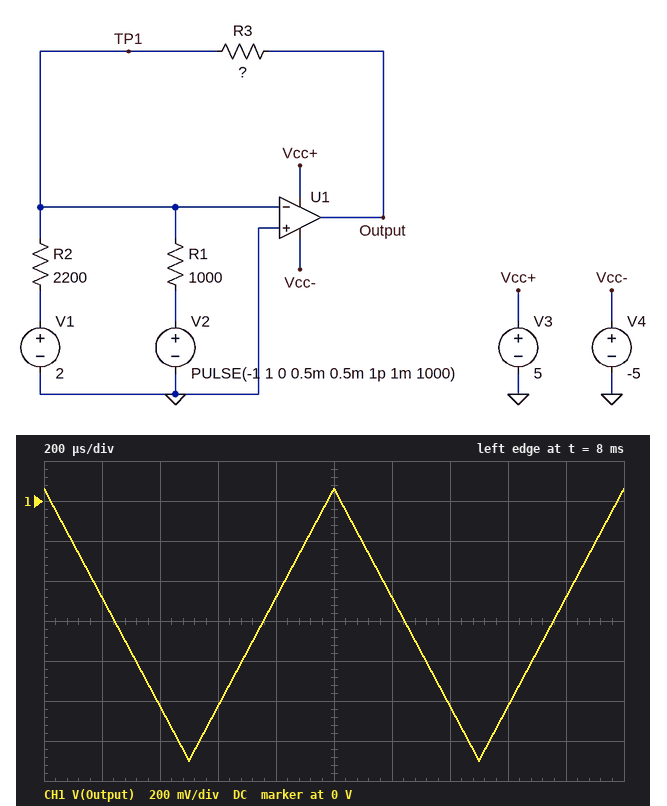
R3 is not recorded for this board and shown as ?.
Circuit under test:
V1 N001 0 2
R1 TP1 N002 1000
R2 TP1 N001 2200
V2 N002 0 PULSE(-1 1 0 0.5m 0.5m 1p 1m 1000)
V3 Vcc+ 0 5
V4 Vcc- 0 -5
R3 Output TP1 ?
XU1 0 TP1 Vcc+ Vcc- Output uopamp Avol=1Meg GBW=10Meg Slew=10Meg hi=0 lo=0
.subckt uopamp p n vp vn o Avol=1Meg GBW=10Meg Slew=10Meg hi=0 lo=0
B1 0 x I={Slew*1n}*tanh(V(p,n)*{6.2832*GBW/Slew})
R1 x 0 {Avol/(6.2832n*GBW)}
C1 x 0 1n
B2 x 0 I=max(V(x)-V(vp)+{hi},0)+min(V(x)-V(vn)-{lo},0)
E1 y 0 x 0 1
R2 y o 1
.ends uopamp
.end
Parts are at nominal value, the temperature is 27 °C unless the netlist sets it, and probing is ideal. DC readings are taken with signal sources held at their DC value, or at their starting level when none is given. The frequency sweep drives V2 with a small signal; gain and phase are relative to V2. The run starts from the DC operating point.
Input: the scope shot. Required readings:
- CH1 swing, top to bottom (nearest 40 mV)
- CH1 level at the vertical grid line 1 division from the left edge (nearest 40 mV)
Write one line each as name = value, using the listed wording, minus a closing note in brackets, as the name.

CH1 swing, top to bottom = 1.36 V
CH1 level at the vertical grid line 1 division from the left edge = -480 mV
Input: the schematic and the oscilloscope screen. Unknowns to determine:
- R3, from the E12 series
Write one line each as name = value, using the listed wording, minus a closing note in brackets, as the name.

R3, from the E12 series = 680 Ω
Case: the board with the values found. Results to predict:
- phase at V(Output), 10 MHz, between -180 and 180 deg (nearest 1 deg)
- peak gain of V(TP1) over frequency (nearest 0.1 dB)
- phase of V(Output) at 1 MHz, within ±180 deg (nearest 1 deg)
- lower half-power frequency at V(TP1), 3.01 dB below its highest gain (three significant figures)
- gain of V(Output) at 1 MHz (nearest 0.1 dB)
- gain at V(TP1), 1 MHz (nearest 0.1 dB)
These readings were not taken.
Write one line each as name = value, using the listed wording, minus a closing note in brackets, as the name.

phase at V(Output), 10 MHz, between -180 and 180 deg = 117 deg
peak gain of V(TP1) over frequency = -9.3 dB
phase of V(Output) at 1 MHz, within ±180 deg = 169 deg
lower half-power frequency at V(TP1), 3.01 dB below its highest gain = 5.02 MHz
gain of V(Output) at 1 MHz = -3.5 dB
gain at V(TP1), 1 MHz = -23.5 dB
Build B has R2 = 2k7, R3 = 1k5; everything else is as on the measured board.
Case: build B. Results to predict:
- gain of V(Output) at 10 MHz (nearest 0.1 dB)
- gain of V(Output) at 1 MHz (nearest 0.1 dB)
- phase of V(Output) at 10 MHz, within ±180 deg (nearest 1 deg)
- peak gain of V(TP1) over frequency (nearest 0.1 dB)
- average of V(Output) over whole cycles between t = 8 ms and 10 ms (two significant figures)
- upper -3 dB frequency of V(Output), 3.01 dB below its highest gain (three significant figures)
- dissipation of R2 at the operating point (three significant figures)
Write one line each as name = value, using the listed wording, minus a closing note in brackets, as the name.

gain of V(Output) at 10 MHz = -6.6 dB
gain of V(Output) at 1 MHz = 3.1 dB
phase of V(Output) at 10 MHz, within ±180 deg = 108 deg
peak gain of V(TP1) over frequency = -6.2 dB
average of V(Output) over whole cycles between t = 8 ms and 10 ms = -1.1 V
upper -3 dB frequency of V(Output), 3.01 dB below its highest gain = 3.27 MHz
dissipation of R2 at the operating point = 1.48 mW
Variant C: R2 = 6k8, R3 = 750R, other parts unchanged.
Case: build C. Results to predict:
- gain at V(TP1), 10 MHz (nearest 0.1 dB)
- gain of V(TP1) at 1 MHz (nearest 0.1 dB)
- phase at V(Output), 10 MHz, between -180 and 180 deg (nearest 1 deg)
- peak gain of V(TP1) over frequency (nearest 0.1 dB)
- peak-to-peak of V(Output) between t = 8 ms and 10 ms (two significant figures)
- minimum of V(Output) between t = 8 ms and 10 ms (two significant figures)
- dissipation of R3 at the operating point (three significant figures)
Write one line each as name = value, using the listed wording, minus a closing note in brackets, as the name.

gain at V(TP1), 10 MHz = -9.0 dB
gain of V(TP1) at 1 MHz = -22.6 dB
phase at V(Output), 10 MHz, between -180 and 180 deg = 118 deg
peak gain of V(TP1) over frequency = -7.9 dB
peak-to-peak of V(Output) between t = 8 ms and 10 ms = 1.5 V
minimum of V(Output) between t = 8 ms and 10 ms = -970 mV
dissipation of R3 at the operating point = 374 µW
